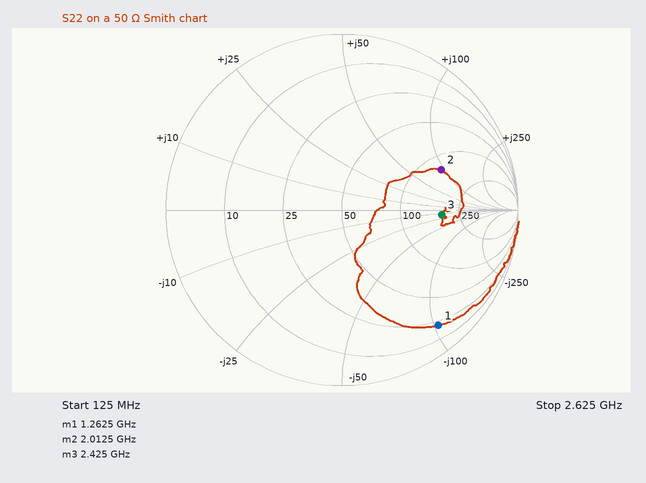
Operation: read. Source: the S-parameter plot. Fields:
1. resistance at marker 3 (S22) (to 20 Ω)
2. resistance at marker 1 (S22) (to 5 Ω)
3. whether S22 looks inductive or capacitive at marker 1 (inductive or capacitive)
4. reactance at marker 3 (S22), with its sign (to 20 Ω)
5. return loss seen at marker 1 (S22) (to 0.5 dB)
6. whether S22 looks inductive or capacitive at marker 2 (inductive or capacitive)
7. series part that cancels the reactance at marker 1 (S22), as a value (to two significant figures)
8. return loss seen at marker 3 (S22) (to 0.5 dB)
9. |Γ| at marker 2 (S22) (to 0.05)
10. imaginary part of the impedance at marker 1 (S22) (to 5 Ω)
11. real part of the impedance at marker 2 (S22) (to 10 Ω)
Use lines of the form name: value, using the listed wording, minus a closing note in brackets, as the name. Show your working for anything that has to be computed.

resistance at marker 3 (S22): 180 Ω
resistance at marker 1 (S22): 20 Ω
whether S22 looks inductive or capacitive at marker 1: capacitive
reactance at marker 3 (S22), with its sign: -20 Ω
return loss seen at marker 1 (S22): 1.5 dB
whether S22 looks inductive or capacitive at marker 2: inductive
series part that cancels the reactance at marker 1 (S22), as a value: L = 105 Ω/(2π × 1.2625 GHz) ≈ 13 nH
return loss seen at marker 3 (S22): 5.0 dB
|Γ| at marker 2 (S22): 0.60
imaginary part of the impedance at marker 1 (S22): -105 Ω
real part of the impedance at marker 2 (S22): 130 Ω
